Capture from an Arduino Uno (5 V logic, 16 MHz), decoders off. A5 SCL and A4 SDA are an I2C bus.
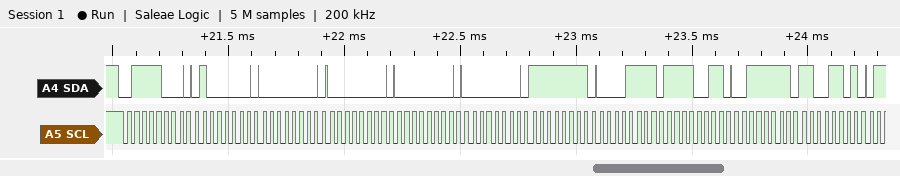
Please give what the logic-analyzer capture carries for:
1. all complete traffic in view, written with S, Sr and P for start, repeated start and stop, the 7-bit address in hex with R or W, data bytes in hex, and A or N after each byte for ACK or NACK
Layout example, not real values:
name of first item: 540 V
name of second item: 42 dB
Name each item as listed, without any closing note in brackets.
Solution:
all complete traffic in view, written with S, Sr and P for start, repeated start and stop, the 7-bit address in hex with R or W, data bytes in hex, and A or N after each byte for ACK or NACK: S 3CW A 40 A 00 A 00 A 00 A 00 A FF A 0F A F3 A 3F A CD A
